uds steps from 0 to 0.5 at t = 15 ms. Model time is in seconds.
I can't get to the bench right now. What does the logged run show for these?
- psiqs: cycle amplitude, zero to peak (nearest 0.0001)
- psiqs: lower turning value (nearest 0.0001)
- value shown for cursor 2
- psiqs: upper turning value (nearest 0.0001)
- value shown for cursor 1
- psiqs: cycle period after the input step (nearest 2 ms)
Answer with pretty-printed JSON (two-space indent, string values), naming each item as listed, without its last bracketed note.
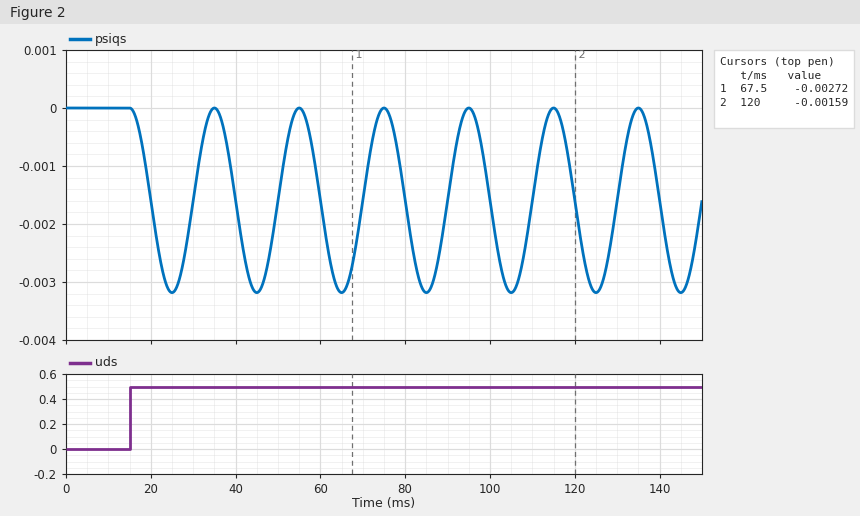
{
  "psiqs: cycle amplitude, zero to peak": "0.0016",
  "psiqs: lower turning value": "-0.0032",
  "value shown for cursor 2": "-0.00159",
  "psiqs: upper turning value": "0.0000",
  "value shown for cursor 1": "-0.00272",
  "psiqs: cycle period after the input step": "20 ms"
}
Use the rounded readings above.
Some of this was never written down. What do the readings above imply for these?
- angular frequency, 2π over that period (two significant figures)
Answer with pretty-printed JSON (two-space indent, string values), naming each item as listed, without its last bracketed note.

{
  "angular frequency, 2π over that period": "0.31 rad/ms"
}
